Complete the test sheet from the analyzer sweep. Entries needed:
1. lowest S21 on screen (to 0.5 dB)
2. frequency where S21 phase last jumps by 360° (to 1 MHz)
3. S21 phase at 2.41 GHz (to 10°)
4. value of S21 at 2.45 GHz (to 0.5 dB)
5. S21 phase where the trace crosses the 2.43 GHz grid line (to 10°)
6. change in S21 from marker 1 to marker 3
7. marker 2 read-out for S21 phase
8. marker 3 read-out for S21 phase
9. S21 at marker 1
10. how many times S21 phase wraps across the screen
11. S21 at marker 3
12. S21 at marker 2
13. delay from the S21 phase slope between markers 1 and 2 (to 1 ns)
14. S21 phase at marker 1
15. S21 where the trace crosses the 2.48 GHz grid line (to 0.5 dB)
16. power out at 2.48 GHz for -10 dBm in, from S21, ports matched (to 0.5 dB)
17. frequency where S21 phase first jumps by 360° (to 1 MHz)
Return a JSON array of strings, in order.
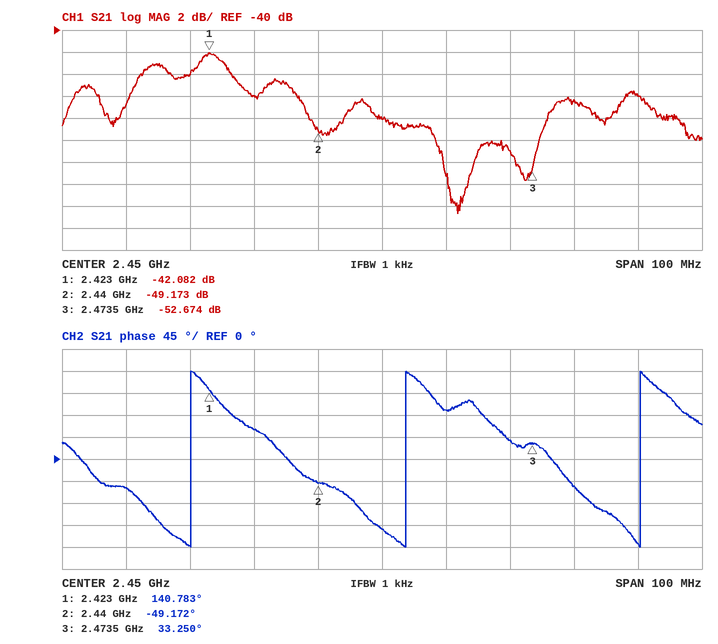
["-56.5 dB", "2.490 GHz", "-60°", "-48.0 dB", "60°", "-10.592 dB", "-49.172°", "33.250°", "-42.082 dB", "3", "-52.674 dB", "-49.173 dB", "31 ns", "140.783°", "-46.5 dB", "-56.5 dBm", "2.420 GHz"]
